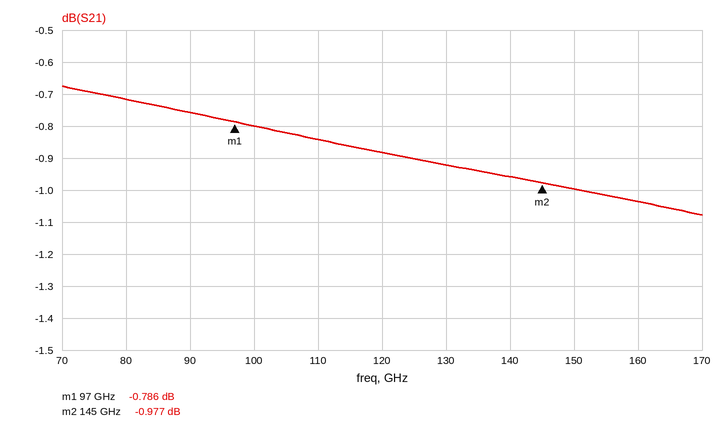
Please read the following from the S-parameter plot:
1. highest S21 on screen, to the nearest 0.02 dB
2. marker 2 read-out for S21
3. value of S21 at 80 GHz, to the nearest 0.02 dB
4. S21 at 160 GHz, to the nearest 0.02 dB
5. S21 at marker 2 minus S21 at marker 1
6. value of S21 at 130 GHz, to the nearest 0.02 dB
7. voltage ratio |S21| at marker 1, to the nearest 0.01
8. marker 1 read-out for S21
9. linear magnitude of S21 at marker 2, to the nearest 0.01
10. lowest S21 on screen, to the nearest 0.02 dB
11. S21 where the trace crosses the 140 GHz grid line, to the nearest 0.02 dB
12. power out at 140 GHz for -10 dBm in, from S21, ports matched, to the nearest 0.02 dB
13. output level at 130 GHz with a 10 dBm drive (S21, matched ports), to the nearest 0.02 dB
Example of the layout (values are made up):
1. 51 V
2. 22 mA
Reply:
1. -0.68 dB
2. -0.977 dB
3. -0.72 dB
4. -1.04 dB
5. -0.191 dB
6. -0.92 dB
7. 0.91
8. -0.786 dB
9. 0.89
10. -1.08 dB
11. -0.96 dB
12. -10.96 dBm
13. 9.08 dBm
